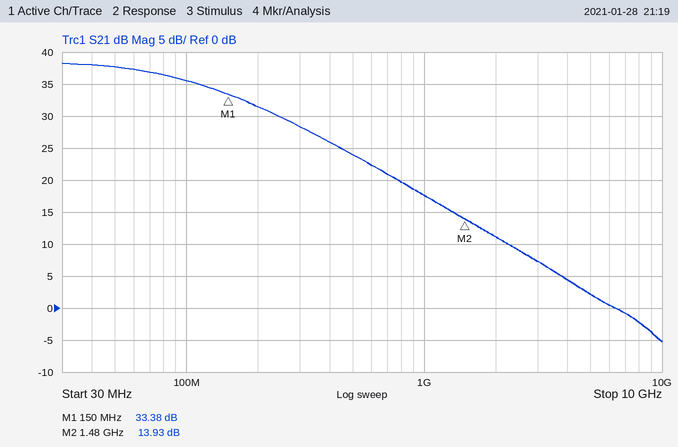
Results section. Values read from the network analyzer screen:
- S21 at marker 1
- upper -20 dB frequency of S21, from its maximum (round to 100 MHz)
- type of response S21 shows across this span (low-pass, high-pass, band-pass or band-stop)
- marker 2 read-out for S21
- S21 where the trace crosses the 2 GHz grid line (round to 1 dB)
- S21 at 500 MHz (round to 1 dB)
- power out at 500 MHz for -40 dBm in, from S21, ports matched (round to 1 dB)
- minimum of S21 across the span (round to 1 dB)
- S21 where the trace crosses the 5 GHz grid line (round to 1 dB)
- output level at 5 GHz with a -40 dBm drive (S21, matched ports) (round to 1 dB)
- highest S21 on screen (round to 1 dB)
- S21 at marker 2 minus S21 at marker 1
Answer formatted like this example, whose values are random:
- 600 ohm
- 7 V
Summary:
- 33.38 dB
- 900 MHz
- low-pass
- 13.93 dB
- 11 dB
- 24 dB
- -16 dBm
- -5 dB
- 2 dB
- -38 dBm
- 38 dB
- -19.45 dB
